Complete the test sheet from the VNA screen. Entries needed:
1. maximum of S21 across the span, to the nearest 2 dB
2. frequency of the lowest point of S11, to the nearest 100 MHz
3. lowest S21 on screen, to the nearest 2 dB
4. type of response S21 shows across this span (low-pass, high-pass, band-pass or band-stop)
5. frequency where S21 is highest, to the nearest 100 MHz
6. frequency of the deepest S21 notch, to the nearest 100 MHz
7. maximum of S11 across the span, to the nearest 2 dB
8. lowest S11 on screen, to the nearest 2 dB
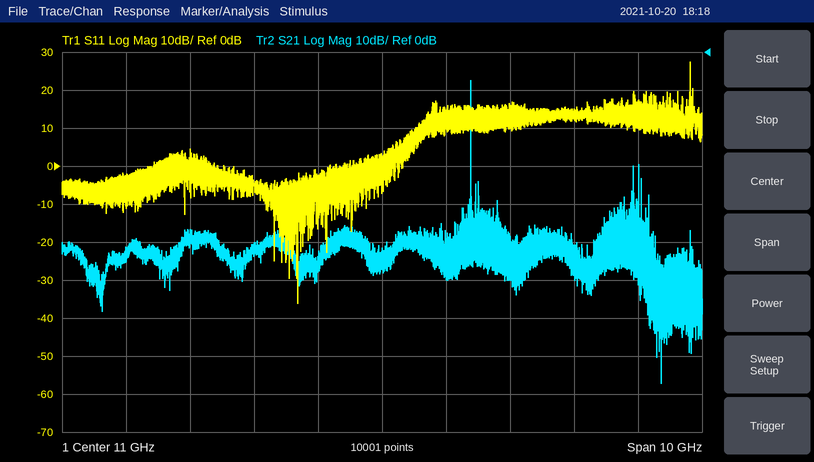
-8 dB
9.7 GHz
-88 dB
band-pass
12.4 GHz
15.4 GHz
28 dB
-36 dB
